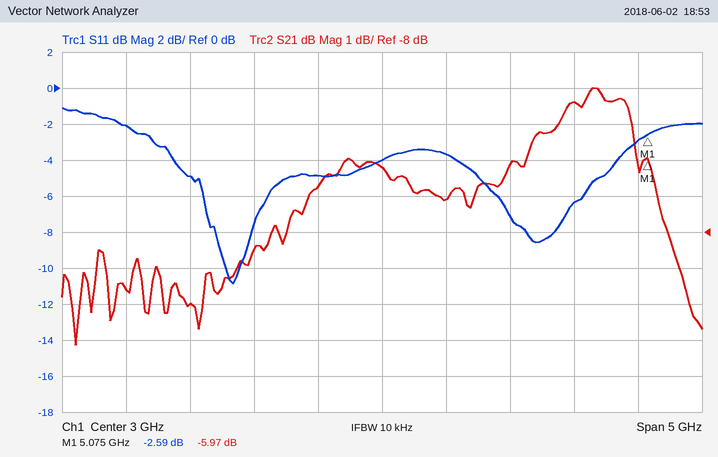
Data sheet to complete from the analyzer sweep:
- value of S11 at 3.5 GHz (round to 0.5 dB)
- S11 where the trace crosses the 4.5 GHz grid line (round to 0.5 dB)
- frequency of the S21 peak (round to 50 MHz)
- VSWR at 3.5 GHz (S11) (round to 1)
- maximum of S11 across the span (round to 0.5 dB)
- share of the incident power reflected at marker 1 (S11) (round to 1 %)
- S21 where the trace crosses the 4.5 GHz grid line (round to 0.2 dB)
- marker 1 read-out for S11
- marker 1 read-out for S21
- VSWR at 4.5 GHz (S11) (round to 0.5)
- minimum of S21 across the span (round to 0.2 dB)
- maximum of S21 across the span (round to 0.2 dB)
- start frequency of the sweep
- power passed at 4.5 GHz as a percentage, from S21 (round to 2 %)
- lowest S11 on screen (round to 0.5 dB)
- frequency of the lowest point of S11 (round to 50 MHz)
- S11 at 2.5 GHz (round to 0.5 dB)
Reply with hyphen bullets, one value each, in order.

- -3.5 dB
- -6.5 dB
- 4.65 GHz
- 5
- -1.0 dB
- 55 %
- -4.4 dB
- -2.59 dB
- -5.97 dB
- 3.0
- -11.2 dB
- -4.0 dB
- 500 MHz
- 36 %
- -11.0 dB
- 1.85 GHz
- -5.0 dB
